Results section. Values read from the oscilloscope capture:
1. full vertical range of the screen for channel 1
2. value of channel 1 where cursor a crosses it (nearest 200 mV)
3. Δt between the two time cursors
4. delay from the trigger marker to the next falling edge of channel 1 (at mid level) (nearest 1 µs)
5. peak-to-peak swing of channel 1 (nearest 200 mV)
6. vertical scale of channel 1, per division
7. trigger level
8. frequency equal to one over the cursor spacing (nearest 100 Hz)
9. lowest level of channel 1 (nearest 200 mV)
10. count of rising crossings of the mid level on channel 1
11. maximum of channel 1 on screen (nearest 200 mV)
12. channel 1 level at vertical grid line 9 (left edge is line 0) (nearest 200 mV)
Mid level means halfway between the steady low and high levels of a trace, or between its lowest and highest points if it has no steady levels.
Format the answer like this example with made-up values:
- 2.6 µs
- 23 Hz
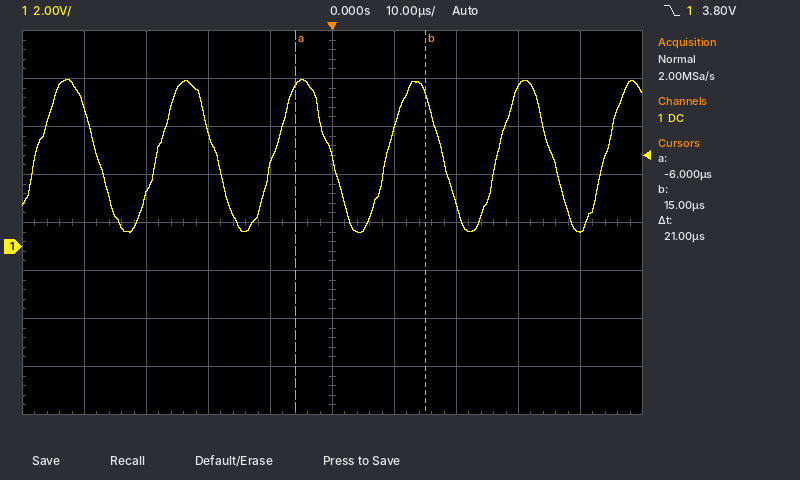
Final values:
- 16 V
- 6.6 V
- 21 µs
- 18 µs
- 6.4 V
- 2 V
- 3.80 V
- 47.6 kHz
- 600 mV
- 6
- 7.0 V
- 600 mV
